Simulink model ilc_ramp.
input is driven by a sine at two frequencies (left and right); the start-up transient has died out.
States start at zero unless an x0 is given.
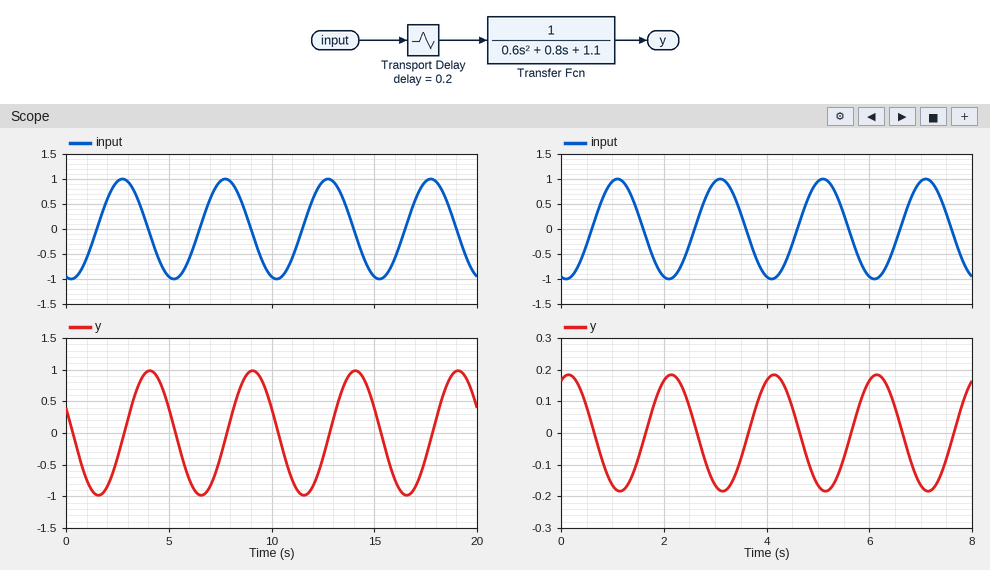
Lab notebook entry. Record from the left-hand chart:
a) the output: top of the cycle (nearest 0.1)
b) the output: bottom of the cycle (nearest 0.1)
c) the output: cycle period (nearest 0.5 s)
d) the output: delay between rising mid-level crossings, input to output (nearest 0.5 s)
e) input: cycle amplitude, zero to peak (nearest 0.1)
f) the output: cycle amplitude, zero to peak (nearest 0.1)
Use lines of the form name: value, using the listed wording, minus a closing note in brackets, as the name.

the output: top of the cycle: 1.0
the output: bottom of the cycle: -1.0
the output: cycle period: 5.0 s
the output: delay between rising mid-level crossings, input to output: 1.5 s
input: cycle amplitude, zero to peak: 1.0
the output: cycle amplitude, zero to peak: 1.0
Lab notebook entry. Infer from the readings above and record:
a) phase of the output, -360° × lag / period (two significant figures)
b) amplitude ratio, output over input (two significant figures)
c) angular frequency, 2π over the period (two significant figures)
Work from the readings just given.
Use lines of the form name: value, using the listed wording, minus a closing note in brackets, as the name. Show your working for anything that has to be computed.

phase of the output, -360° × lag / period: -360 × 1.5 / 5 = -110°
amplitude ratio, output over input: 1 / 1 = 1.0
angular frequency, 2π over the period: 2π / 5 = 1.3 rad/s
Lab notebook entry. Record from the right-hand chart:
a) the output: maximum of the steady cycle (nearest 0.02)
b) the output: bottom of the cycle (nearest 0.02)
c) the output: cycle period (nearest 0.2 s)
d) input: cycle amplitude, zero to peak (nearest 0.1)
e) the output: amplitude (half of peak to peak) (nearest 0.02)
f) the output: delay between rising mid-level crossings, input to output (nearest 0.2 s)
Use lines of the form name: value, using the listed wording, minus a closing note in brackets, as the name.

the output: maximum of the steady cycle: 0.18
the output: bottom of the cycle: -0.18
the output: cycle period: 2.0 s
input: cycle amplitude, zero to peak: 1.0
the output: amplitude (half of peak to peak): 0.18
the output: delay between rising mid-level crossings, input to output: 1.0 s
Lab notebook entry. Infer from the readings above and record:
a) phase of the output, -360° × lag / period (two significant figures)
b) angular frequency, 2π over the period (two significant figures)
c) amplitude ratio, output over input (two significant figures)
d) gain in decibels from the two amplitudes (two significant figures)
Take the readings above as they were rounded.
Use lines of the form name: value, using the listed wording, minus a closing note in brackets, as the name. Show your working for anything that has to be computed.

phase of the output, -360° × lag / period: -360 × 1 / 2 = -180°
angular frequency, 2π over the period: 2π / 2 = 3.1 rad/s
amplitude ratio, output over input: 0.18 / 1 = 0.18
gain in decibels from the two amplitudes: 20 log10(0.18 / 1) = -15 dB
